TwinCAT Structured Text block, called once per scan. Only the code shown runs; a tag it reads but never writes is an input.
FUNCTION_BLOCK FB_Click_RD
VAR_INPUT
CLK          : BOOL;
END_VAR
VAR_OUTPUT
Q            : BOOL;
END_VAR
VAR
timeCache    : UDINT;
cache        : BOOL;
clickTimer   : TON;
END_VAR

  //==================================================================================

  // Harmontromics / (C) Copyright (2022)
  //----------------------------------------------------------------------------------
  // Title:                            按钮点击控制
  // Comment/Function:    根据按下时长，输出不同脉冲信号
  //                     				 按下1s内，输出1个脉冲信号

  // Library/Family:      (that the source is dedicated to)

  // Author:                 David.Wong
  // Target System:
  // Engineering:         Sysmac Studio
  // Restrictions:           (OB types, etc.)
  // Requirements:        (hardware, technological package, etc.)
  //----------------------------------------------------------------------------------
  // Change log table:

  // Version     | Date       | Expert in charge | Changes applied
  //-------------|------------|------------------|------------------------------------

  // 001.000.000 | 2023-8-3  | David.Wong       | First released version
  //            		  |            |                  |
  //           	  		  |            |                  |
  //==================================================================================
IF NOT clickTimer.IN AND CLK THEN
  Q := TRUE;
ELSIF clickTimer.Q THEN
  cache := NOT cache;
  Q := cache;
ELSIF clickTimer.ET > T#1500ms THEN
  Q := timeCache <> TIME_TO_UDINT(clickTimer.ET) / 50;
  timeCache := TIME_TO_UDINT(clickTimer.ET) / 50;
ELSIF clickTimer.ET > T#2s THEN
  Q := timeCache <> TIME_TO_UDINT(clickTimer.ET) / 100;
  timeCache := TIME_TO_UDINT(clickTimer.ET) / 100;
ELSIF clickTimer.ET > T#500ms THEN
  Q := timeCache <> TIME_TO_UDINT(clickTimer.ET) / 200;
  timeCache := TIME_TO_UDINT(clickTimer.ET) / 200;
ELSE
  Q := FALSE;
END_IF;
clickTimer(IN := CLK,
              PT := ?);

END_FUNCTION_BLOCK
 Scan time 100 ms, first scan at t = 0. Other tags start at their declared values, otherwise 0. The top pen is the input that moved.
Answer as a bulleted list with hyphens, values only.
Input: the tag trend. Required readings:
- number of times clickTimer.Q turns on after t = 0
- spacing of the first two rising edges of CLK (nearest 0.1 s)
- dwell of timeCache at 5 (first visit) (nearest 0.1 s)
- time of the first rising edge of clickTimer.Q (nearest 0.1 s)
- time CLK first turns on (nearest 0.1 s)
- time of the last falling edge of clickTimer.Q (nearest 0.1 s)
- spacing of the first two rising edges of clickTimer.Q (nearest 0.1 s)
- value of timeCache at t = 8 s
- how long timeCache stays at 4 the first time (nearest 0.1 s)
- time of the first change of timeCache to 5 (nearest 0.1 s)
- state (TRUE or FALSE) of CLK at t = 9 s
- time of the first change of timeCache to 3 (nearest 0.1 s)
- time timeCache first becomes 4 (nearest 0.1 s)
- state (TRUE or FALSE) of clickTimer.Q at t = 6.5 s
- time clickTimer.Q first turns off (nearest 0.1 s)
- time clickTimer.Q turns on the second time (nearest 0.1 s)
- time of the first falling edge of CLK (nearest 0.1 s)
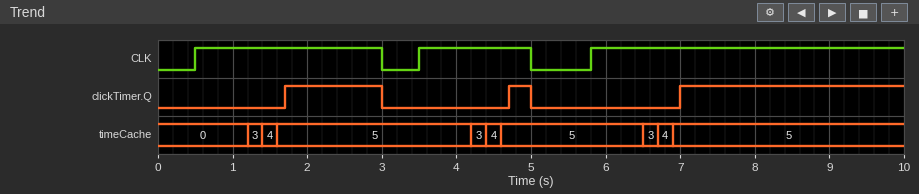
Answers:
- 3
- 3.0 s
- 2.6 s
- 1.7 s
- 0.5 s
- 5.0 s
- 3.0 s
- 5
- 0.2 s
- 1.6 s
- TRUE
- 1.2 s
- 1.4 s
- FALSE
- 3.0 s
- 4.7 s
- 3.0 s
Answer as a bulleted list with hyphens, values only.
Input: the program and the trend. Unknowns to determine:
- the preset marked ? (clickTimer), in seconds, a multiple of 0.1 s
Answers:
- 1.2 s
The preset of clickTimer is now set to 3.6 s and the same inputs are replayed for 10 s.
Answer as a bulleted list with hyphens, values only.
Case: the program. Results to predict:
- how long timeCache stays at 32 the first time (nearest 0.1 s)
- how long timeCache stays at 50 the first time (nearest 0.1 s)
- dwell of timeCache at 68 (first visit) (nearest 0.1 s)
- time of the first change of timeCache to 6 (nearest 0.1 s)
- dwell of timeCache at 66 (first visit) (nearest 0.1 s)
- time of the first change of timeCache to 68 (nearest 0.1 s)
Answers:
- 0.1 s
- 0.1 s
- 0.1 s
- 1.8 s
- 0.1 s
- 9.3 s
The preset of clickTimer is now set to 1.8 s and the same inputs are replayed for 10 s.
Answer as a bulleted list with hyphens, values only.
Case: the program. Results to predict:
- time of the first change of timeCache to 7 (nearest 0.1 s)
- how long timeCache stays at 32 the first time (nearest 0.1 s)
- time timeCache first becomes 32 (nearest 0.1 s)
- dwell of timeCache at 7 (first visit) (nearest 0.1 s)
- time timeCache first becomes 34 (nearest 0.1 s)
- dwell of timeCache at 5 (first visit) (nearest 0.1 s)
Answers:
- 2.0 s
- 0.1 s
- 2.2 s
- 0.2 s
- 2.3 s
- 0.2 s
